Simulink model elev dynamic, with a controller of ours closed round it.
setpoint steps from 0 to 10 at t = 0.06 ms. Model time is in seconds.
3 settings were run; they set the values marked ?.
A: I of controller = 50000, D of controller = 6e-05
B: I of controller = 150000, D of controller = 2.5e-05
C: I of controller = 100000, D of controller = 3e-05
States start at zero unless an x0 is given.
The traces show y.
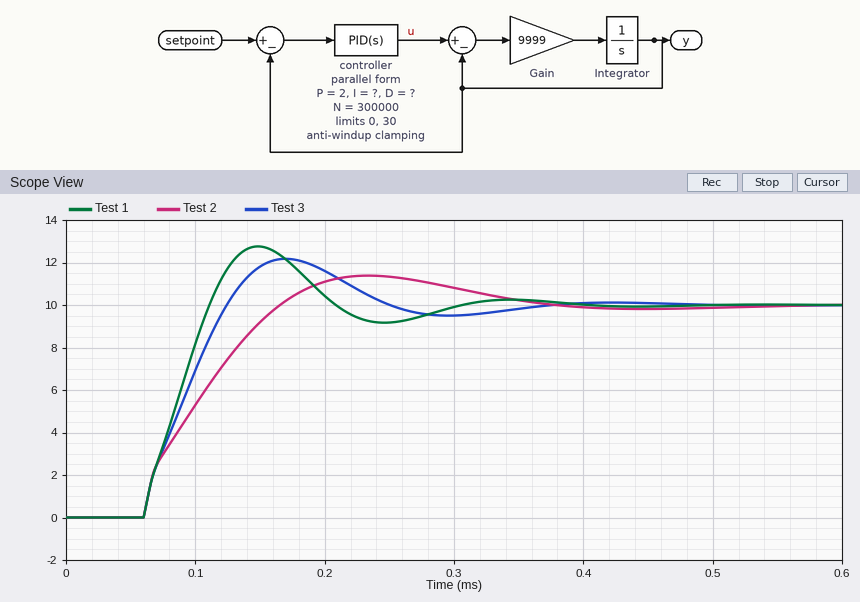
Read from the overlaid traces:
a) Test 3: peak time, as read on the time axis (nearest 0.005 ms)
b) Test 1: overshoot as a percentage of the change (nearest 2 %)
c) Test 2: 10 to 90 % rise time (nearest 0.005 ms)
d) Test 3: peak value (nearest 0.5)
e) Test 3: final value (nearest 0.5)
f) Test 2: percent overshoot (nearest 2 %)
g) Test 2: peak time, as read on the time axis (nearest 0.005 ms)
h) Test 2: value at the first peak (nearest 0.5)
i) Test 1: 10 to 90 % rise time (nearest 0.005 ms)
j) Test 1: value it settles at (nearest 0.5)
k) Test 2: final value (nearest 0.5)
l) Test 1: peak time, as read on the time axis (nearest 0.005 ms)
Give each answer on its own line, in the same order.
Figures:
0.170 ms
28 %
0.085 ms
12.0
10.0
14 %
0.235 ms
11.5
0.040 ms
10.0
10.0
0.150 ms
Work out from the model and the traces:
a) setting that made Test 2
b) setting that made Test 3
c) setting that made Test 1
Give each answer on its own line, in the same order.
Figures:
A
C
B
